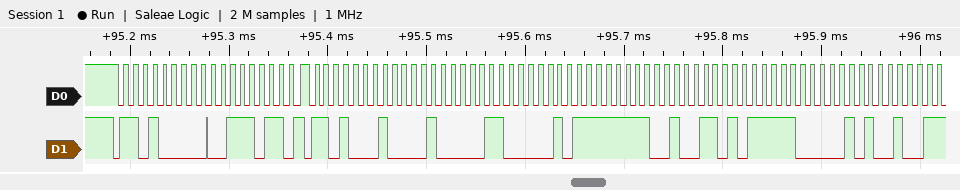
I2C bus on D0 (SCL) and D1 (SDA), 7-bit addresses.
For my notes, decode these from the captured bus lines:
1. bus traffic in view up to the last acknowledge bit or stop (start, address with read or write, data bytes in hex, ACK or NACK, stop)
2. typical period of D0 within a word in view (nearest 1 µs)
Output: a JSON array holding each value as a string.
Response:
["start, address 68 write ACK, 3B ACK, repeated start, address 68 read ACK, 10 ACK, C1 ACK, FF ACK, 4D ACK, F8 ACK, 52 ACK", "10 µs"]
